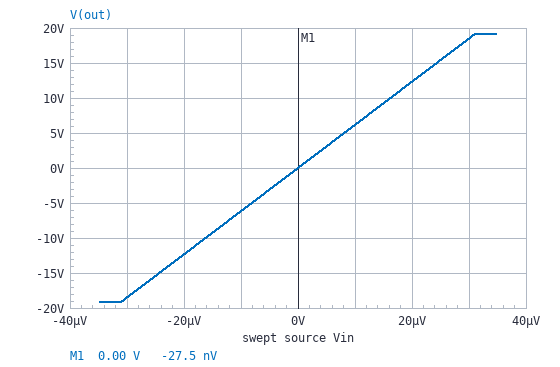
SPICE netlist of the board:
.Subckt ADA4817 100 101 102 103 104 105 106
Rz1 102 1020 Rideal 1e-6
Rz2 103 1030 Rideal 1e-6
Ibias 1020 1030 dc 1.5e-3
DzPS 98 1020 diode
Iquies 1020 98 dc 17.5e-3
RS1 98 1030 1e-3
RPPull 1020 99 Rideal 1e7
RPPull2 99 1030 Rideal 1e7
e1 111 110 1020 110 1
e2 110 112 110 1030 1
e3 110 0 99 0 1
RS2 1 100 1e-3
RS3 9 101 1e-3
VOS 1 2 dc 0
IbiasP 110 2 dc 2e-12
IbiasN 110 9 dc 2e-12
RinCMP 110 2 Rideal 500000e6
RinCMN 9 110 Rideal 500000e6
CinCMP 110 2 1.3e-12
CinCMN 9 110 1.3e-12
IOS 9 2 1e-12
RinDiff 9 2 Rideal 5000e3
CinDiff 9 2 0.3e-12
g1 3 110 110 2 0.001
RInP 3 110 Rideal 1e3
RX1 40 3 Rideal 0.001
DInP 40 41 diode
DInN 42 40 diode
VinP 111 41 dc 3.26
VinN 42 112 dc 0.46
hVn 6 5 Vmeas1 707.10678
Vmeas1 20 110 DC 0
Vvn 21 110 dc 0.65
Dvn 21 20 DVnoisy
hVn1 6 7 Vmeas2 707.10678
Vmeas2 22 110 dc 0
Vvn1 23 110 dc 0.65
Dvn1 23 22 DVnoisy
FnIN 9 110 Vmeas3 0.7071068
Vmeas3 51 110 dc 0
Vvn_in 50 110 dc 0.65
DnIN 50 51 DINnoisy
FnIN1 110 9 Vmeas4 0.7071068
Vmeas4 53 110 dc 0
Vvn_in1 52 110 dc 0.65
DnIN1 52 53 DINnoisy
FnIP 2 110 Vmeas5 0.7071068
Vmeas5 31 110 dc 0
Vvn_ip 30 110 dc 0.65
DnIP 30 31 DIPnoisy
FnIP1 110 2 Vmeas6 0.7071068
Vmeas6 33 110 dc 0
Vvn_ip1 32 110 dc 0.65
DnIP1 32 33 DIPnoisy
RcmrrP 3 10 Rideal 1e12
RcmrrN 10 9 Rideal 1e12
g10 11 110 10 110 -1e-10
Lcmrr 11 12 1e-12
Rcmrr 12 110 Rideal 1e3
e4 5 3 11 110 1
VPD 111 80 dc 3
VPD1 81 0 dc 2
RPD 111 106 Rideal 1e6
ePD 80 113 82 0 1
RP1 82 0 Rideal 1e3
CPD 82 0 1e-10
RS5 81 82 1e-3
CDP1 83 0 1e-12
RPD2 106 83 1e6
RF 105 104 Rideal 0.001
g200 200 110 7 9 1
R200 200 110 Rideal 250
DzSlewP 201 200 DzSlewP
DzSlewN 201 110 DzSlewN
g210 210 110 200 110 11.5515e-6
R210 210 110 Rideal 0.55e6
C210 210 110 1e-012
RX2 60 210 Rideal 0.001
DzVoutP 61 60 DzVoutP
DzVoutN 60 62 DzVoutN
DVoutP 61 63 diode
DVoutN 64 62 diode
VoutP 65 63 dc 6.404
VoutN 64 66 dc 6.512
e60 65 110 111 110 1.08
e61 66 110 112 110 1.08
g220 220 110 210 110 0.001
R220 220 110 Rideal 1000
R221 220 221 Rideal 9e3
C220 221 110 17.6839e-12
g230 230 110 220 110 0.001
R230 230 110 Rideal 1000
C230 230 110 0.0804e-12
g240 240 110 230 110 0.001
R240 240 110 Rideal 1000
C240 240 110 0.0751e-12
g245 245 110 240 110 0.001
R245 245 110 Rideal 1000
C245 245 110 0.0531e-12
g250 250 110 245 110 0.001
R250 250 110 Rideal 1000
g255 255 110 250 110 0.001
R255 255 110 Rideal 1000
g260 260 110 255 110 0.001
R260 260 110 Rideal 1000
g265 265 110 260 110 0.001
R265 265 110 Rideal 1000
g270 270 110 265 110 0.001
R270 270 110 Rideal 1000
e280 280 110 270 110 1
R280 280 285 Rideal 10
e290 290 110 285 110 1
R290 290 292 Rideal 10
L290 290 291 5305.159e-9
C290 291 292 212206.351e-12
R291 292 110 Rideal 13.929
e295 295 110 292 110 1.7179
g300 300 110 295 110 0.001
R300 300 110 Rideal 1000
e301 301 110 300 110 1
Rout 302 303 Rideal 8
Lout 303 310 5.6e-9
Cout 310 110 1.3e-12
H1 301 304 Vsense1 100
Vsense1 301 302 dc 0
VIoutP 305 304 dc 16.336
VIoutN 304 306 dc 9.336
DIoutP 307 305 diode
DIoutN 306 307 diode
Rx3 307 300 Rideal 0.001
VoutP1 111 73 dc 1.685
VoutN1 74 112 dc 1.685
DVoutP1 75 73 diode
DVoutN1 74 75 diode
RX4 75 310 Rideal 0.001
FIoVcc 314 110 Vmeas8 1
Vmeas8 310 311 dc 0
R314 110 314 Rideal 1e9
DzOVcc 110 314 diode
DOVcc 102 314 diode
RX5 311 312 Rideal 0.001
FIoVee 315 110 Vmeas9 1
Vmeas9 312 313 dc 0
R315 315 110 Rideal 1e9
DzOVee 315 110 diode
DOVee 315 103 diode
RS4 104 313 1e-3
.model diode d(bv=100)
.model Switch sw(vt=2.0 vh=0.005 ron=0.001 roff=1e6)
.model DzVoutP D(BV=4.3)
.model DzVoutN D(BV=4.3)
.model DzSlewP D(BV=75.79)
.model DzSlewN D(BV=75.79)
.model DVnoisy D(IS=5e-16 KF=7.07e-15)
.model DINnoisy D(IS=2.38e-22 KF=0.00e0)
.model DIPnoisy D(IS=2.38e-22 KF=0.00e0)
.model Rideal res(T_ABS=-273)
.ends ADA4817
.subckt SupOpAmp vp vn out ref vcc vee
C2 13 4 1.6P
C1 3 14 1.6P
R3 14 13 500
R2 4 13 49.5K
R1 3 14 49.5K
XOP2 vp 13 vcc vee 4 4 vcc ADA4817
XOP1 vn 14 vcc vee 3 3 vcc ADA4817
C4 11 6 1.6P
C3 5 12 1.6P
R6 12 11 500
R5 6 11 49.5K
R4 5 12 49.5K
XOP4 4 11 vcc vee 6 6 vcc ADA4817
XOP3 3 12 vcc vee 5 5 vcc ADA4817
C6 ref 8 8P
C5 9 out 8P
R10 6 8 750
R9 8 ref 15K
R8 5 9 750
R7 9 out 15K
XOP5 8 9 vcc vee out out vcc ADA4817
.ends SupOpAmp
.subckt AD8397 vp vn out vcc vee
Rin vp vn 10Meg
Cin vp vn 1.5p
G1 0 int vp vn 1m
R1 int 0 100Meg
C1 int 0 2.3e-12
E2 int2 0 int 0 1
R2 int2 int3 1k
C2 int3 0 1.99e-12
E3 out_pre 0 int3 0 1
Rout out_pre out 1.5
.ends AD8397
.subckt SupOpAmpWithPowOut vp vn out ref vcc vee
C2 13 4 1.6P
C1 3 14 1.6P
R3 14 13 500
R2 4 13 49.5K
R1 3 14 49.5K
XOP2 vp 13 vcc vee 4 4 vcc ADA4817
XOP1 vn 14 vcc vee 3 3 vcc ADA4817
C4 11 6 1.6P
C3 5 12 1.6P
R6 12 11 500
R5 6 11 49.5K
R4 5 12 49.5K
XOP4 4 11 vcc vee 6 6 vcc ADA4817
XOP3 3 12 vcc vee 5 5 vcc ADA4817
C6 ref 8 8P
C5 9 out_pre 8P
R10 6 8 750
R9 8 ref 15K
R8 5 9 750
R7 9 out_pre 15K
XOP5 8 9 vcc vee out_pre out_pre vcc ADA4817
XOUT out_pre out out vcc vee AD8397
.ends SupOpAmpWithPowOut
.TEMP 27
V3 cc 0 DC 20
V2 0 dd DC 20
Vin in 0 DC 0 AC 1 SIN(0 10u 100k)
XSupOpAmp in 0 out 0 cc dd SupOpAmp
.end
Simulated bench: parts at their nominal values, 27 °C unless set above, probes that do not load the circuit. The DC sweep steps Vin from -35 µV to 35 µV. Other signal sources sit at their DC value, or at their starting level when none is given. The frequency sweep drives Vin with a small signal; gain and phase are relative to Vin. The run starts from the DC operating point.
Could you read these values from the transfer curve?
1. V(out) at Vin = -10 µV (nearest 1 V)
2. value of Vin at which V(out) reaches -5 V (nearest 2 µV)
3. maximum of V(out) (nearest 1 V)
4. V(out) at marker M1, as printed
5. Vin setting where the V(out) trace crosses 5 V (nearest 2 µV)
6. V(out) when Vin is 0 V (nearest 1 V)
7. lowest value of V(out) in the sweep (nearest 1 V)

-6 V
-8 µV
19 V
-27.5 nV
8 µV
0 V
-19 V
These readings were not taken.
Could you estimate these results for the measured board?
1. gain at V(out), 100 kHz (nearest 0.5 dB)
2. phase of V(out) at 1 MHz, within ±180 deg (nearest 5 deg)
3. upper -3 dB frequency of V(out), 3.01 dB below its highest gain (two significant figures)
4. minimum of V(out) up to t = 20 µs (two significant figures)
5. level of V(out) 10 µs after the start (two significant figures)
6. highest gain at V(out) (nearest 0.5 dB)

116.5 dB
-125 deg
640 kHz
-6.6 V
-1.2 V
116.5 dB
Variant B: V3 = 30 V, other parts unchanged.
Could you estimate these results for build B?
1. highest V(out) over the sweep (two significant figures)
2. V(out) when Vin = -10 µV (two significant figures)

22 V
-6.1 V
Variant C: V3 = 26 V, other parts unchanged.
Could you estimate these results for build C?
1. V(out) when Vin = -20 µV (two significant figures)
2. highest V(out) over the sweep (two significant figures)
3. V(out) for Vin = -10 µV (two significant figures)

-12 V
22 V
-6.1 V
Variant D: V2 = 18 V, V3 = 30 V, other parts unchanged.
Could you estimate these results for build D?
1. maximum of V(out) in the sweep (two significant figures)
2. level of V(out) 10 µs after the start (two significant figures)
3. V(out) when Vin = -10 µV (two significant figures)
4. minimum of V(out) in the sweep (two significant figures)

22 V
-1.1 V
-6.1 V
-17 V
